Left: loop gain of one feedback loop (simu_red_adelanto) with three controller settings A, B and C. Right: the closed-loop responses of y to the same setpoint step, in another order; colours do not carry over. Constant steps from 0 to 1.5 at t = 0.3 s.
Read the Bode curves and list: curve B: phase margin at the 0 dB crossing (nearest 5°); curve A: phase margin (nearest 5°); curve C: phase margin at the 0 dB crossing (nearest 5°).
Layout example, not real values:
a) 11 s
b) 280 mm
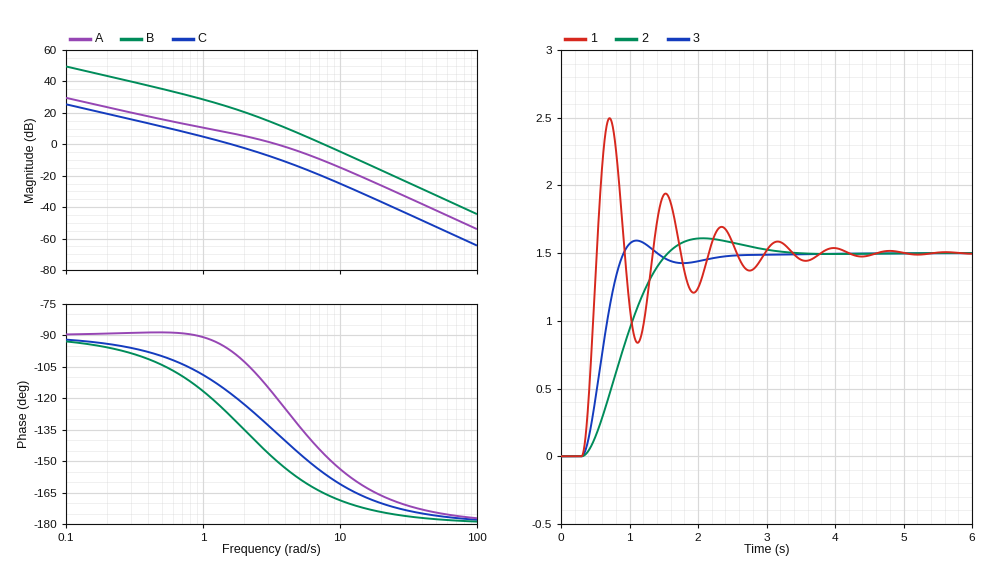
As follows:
a) 15°
b) 60°
c) 60°
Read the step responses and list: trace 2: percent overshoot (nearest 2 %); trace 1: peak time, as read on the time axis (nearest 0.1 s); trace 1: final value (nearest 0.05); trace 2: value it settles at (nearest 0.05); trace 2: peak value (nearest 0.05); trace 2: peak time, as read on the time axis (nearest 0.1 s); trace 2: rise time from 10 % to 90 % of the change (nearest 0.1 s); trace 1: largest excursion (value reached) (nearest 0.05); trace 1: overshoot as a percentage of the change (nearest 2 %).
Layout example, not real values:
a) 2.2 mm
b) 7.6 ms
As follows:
a) 8 %
b) 0.7 s
c) 1.50
d) 1.50
e) 1.60
f) 2.1 s
g) 0.8 s
h) 2.50
i) 66 %
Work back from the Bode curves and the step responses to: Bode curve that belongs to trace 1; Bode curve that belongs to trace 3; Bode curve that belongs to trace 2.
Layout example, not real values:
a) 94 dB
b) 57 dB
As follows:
a) B
b) A
c) C
